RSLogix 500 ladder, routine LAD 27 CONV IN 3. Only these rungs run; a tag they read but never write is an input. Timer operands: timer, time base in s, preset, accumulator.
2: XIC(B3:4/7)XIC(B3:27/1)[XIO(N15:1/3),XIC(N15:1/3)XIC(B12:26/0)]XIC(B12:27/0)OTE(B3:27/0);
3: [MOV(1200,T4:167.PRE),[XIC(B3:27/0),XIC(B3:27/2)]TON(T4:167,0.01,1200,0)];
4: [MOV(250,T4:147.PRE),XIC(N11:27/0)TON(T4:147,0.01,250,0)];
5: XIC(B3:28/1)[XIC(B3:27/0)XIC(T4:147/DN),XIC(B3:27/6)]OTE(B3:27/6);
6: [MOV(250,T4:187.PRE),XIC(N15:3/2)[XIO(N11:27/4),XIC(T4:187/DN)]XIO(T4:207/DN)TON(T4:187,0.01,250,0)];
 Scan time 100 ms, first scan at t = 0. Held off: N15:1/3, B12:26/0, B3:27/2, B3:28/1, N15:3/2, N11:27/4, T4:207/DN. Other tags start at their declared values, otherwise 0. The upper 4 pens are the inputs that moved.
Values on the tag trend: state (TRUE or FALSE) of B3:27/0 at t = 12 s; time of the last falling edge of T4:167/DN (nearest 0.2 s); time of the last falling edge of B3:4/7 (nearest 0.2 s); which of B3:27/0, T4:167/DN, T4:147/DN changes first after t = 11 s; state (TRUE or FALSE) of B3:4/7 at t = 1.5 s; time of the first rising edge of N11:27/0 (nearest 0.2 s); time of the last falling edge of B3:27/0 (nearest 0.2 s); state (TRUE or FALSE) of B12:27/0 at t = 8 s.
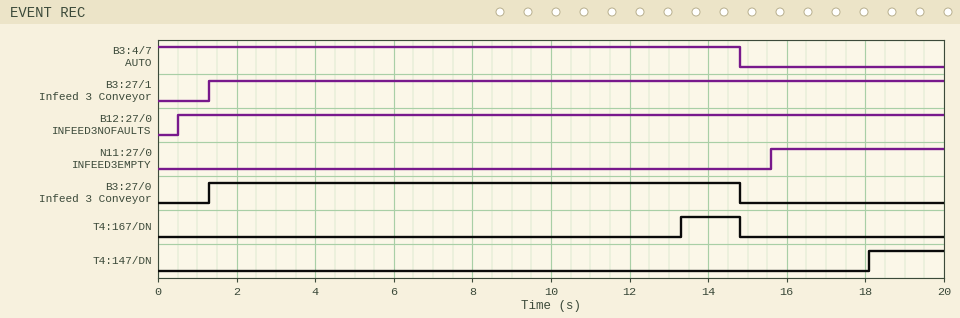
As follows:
TRUE
14.8 s
14.8 s
T4:167/DN
TRUE
15.6 s
14.8 s
TRUE
